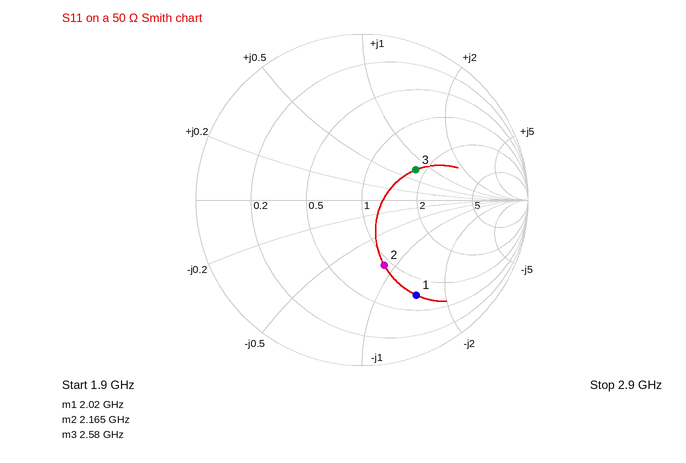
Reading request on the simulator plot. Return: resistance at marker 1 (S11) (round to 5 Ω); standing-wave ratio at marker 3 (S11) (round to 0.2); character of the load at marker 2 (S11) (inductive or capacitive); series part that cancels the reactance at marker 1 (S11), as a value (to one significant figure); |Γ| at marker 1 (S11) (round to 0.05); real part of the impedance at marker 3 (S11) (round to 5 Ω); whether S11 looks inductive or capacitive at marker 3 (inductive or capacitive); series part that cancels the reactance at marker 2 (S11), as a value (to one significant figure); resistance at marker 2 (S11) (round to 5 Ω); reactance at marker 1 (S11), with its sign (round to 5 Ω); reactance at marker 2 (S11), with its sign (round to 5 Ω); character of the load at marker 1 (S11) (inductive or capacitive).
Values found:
35 Ω
2.2
capacitive
6 nH
0.65
90 Ω
inductive
3 nH
45 Ω
-75 Ω
-45 Ω
capacitive
